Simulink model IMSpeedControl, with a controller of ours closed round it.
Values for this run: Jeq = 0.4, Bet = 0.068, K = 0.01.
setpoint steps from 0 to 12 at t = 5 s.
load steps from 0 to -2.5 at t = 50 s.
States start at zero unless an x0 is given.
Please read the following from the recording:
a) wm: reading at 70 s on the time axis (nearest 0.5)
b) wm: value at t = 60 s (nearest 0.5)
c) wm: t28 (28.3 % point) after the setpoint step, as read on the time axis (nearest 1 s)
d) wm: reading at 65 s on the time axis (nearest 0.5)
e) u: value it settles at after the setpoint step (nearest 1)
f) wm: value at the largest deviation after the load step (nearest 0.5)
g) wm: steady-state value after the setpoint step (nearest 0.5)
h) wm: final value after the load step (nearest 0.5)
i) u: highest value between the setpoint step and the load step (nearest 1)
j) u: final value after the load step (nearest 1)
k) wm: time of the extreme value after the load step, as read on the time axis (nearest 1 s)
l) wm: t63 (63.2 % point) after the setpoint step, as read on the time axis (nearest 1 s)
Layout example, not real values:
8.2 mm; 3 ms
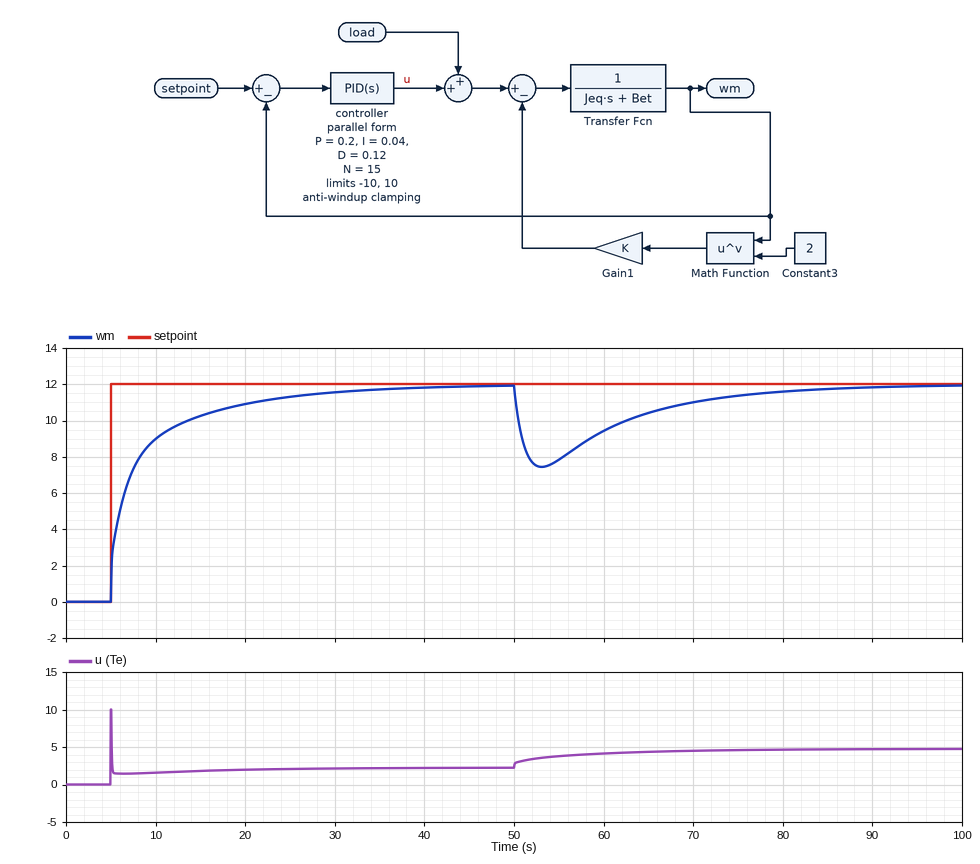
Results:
11.0; 9.5; 5 s; 10.5; 2; 7.5; 12.0; 12.0; 10; 5; 53 s; 8 s
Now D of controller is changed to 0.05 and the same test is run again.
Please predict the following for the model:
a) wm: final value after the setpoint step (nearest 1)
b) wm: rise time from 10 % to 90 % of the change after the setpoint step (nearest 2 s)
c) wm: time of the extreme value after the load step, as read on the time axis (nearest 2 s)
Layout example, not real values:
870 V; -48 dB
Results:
12; 14 s; 52 s
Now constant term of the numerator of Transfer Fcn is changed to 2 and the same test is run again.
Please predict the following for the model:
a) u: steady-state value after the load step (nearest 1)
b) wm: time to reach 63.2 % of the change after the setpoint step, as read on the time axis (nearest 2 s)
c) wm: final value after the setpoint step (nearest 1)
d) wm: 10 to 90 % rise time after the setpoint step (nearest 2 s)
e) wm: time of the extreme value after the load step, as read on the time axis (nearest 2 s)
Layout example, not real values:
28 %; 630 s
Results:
4; 6 s; 12; 12 s; 52 s
